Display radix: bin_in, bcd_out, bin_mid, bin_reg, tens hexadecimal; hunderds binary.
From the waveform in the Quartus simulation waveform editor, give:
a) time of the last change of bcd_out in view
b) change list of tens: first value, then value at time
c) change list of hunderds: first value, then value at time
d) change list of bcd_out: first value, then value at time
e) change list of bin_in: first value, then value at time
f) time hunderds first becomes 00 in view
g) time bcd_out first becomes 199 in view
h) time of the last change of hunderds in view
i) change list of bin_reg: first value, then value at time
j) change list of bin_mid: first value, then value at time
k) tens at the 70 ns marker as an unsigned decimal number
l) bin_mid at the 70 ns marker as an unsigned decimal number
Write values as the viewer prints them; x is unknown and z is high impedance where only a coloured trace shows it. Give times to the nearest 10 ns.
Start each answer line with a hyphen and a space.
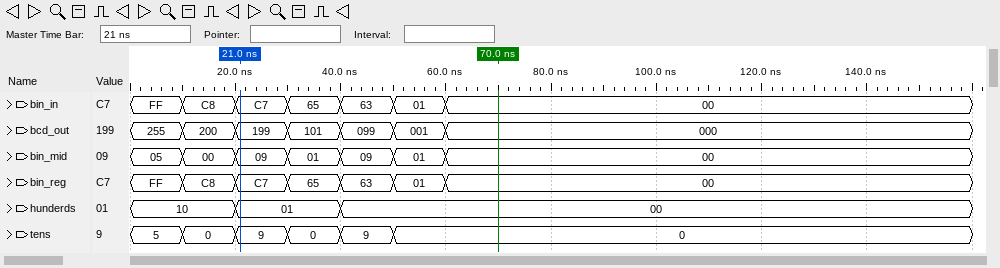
- 60 ns
- 5, 0 at 10 ns, 9 at 20 ns, 0 at 30 ns, 9 at 40 ns, 0 at 50 ns
- 10, 01 at 20 ns, 00 at 40 ns
- 255, 200 at 10 ns, 199 at 20 ns, 101 at 30 ns, 099 at 40 ns, 001 at 50 ns, 000 at 60 ns
- FF, C8 at 10 ns, C7 at 20 ns, 65 at 30 ns, 63 at 40 ns, 01 at 50 ns, 00 at 60 ns
- 40 ns
- 20 ns
- 40 ns
- FF, C8 at 10 ns, C7 at 20 ns, 65 at 30 ns, 63 at 40 ns, 01 at 50 ns, 00 at 60 ns
- 05, 00 at 10 ns, 09 at 20 ns, 01 at 30 ns, 09 at 40 ns, 01 at 50 ns, 00 at 60 ns
- 0
- 0
